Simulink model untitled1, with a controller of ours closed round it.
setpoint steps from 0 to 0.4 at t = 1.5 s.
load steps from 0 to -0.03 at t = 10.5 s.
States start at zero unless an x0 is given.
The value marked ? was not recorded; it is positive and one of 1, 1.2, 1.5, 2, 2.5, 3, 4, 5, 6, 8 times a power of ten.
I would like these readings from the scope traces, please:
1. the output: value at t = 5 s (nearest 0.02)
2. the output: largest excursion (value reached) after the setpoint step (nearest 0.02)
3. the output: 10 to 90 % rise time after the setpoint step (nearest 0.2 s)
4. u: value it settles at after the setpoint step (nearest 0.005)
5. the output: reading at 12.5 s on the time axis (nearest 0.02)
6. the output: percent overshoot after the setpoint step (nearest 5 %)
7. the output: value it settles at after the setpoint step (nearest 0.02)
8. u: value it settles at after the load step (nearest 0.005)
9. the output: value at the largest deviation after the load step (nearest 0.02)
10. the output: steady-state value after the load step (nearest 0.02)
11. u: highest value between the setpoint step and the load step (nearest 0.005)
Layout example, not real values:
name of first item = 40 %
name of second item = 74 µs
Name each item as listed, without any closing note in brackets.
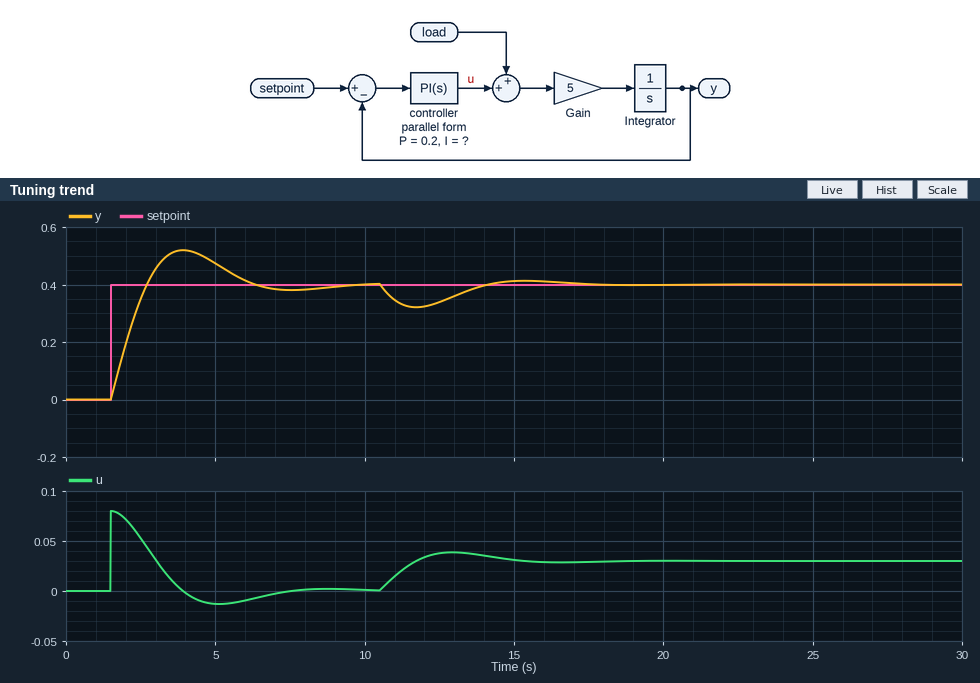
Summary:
the output: value at t = 5 s = 0.48
the output: largest excursion (value reached) after the setpoint step = 0.52
the output: 10 to 90 % rise time after the setpoint step = 1.0 s
u: value it settles at after the setpoint step = 0.000
the output: reading at 12.5 s on the time axis = 0.34
the output: percent overshoot after the setpoint step = 30 %
the output: value it settles at after the setpoint step = 0.40
u: value it settles at after the load step = 0.030
the output: value at the largest deviation after the load step = 0.32
the output: steady-state value after the load step = 0.40
u: highest value between the setpoint step and the load step = 0.080
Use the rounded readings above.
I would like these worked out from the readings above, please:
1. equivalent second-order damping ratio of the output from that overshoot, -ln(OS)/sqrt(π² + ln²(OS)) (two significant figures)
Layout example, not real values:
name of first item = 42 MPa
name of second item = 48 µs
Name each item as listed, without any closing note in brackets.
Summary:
equivalent second-order damping ratio of the output from that overshoot, -ln(OS)/sqrt(π² + ln²(OS)) = 0.36
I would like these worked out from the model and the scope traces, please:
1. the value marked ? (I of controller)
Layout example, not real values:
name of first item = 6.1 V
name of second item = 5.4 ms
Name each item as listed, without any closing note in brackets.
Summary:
the value marked ? = 0.2
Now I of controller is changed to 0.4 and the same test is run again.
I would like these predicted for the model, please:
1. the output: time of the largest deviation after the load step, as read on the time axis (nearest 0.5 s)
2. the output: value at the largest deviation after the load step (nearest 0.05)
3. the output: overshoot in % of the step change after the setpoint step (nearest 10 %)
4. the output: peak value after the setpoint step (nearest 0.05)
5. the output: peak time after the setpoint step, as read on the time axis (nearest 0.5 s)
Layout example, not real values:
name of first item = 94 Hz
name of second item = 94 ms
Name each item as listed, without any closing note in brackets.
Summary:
the output: time of the largest deviation after the load step, as read on the time axis = 11.5 s
the output: value at the largest deviation after the load step = 0.35
the output: overshoot in % of the step change after the setpoint step = 40 %
the output: peak value after the setpoint step = 0.55
the output: peak time after the setpoint step, as read on the time axis = 3.5 s
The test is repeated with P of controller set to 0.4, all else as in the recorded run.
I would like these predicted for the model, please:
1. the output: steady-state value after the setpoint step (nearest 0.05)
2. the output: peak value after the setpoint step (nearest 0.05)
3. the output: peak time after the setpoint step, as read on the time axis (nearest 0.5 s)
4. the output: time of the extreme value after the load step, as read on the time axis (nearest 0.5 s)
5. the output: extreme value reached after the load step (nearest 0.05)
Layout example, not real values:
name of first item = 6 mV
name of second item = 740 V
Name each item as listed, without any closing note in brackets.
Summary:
the output: steady-state value after the setpoint step = 0.40
the output: peak value after the setpoint step = 0.45
the output: peak time after the setpoint step, as read on the time axis = 3.5 s
the output: time of the extreme value after the load step, as read on the time axis = 11.5 s
the output: extreme value reached after the load step = 0.35
